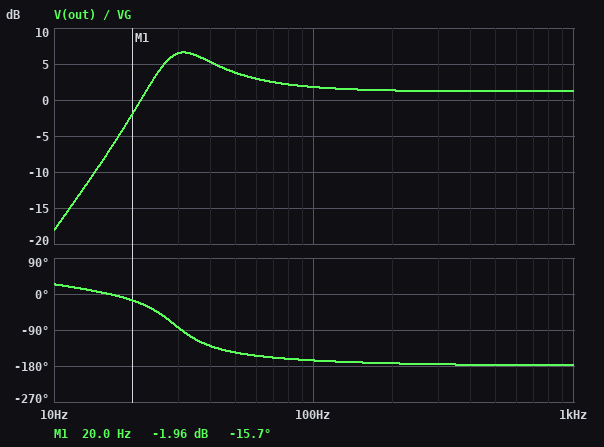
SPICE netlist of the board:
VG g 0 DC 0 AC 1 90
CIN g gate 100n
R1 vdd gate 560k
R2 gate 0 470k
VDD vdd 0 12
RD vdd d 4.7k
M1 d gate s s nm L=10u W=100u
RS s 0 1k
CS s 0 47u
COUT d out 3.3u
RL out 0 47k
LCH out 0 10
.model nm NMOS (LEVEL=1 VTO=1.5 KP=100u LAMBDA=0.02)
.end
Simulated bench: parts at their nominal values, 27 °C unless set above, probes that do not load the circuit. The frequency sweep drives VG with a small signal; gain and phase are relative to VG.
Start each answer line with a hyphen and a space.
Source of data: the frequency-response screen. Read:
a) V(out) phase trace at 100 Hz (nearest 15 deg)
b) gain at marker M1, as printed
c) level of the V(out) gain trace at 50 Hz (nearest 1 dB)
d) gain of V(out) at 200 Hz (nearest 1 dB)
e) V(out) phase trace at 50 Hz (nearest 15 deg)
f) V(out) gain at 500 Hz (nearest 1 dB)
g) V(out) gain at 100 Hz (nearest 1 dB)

- -165 deg
- -1.96 dB
- 4 dB
- 1 dB
- -150 deg
- 1 dB
- 2 dB
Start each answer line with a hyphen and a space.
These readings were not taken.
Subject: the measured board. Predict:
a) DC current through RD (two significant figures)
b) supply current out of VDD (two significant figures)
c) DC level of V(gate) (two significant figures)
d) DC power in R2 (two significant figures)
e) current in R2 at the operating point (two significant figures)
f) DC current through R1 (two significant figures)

- 1.9 mA
- 1.9 mA
- 5.5 V
- 64 µW
- 12 µA
- 12 µA
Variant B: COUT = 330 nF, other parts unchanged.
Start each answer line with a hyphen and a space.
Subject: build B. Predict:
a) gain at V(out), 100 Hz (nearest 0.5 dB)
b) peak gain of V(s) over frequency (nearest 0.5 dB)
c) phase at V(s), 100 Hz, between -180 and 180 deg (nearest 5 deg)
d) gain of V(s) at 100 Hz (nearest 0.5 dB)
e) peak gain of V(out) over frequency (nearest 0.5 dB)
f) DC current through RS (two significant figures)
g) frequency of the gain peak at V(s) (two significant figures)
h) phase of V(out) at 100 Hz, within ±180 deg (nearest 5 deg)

- 10.5 dB
- -22.5 dB
- -105 deg
- -33.0 dB
- 12.5 dB
- 1.9 mA
- 5.5 Hz
- -130 deg
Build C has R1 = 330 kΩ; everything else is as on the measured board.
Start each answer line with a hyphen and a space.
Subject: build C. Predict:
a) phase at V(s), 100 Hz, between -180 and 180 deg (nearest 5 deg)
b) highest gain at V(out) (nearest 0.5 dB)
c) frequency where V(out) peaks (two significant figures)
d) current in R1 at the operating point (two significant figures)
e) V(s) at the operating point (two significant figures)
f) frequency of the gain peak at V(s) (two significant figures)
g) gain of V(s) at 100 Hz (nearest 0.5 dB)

- -115 deg
- -1.5 dB
- 29 Hz
- 15 µA
- 2.0 V
- 28 Hz
- -54.5 dB
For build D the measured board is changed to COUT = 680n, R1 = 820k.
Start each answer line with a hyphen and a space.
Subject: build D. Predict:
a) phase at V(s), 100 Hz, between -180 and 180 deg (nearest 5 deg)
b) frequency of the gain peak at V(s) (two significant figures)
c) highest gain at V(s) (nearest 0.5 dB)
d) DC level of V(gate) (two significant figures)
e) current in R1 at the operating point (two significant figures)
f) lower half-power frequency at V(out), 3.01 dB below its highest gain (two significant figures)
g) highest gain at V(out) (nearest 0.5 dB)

- -85 deg
- 6.8 Hz
- -8.5 dB
- 4.4 V
- 9.3 µA
- 52 Hz
- 17.0 dB
